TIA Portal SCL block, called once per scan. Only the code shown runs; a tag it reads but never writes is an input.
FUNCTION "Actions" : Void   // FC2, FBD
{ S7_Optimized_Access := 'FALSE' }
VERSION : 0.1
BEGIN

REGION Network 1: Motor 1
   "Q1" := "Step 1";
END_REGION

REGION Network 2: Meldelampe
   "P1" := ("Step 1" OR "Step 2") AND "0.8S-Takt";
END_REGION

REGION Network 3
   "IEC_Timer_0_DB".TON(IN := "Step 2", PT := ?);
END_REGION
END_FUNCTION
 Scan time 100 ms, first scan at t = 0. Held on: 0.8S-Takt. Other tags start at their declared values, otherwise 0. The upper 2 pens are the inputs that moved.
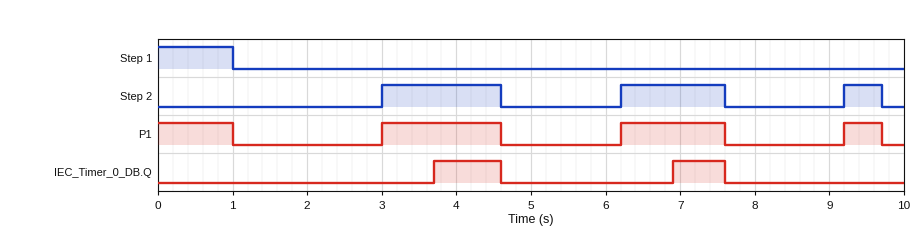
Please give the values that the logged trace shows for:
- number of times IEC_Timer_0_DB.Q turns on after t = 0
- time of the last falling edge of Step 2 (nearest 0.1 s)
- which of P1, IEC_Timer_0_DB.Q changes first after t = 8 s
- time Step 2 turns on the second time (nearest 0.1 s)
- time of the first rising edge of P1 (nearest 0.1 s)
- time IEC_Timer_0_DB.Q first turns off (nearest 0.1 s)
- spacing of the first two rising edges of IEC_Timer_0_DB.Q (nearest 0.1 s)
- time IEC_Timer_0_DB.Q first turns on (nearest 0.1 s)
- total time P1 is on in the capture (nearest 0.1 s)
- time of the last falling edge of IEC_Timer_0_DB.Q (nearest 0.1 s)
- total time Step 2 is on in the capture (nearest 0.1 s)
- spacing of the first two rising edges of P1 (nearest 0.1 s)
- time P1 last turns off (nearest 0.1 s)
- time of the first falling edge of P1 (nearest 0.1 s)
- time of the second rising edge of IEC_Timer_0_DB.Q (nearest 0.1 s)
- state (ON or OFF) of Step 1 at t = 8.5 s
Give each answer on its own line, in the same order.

2
9.7 s
P1
6.2 s
3.0 s
4.6 s
3.2 s
3.7 s
4.5 s
7.6 s
3.5 s
3.2 s
9.7 s
1.0 s
6.9 s
OFF
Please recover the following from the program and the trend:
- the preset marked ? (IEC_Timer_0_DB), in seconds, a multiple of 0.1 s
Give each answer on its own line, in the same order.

0.7 s
